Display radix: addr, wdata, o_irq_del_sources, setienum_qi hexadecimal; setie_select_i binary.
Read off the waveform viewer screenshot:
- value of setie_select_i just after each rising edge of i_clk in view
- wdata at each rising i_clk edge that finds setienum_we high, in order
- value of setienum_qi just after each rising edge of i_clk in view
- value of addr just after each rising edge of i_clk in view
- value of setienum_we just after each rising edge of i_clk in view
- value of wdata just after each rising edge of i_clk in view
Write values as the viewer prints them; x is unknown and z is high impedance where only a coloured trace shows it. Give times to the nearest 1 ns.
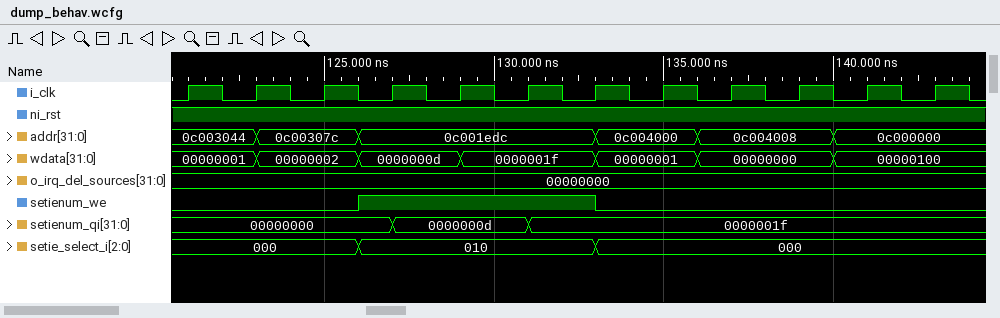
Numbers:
000, 000, 000, 010, 010, 010, 000, 000, 000, 000, 000, 000
0000000d, 0000000d, 0000001f, 0000001f
00000000, 00000000, 00000000, 0000000d, 0000000d, 0000001f, 0000001f, 0000001f, 0000001f, 0000001f, 0000001f, 0000001f
0c003044, 0c00307c, 0c00307c, 0c001edc, 0c001edc, 0c001edc, 0c004000, 0c004000, 0c004008, 0c004008, 0c000000, 0c000000
0 0 0 1 1 1 0 0 0 0 0 0
00000001, 00000002, 00000002, 0000000d, 0000001f, 0000001f, 00000001, 00000001, 00000000, 00000000, 00000100, 00000100
